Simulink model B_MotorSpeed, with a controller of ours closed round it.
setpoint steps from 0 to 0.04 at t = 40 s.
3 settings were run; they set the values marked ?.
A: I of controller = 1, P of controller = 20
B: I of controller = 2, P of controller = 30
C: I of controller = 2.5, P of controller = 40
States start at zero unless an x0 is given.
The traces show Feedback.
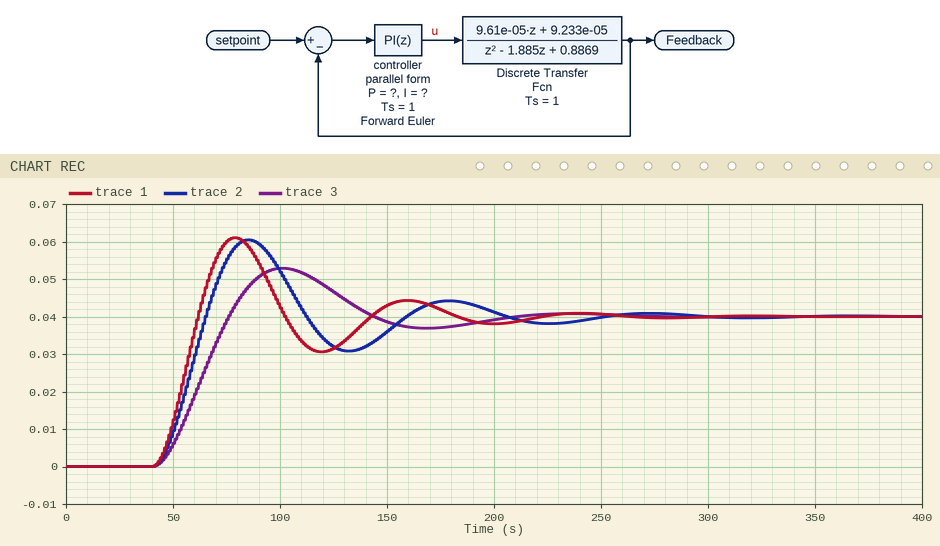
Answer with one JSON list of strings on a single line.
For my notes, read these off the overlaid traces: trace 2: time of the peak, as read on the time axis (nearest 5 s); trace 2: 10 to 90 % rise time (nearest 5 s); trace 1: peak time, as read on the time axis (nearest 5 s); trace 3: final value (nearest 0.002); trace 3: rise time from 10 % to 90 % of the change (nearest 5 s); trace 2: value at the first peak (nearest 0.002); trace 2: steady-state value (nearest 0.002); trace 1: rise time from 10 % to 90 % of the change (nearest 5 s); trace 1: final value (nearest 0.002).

["85 s", "15 s", "80 s", "0.040", "25 s", "0.060", "0.040", "15 s", "0.040"]
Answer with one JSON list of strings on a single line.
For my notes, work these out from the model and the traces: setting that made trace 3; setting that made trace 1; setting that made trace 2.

["A", "C", "B"]
